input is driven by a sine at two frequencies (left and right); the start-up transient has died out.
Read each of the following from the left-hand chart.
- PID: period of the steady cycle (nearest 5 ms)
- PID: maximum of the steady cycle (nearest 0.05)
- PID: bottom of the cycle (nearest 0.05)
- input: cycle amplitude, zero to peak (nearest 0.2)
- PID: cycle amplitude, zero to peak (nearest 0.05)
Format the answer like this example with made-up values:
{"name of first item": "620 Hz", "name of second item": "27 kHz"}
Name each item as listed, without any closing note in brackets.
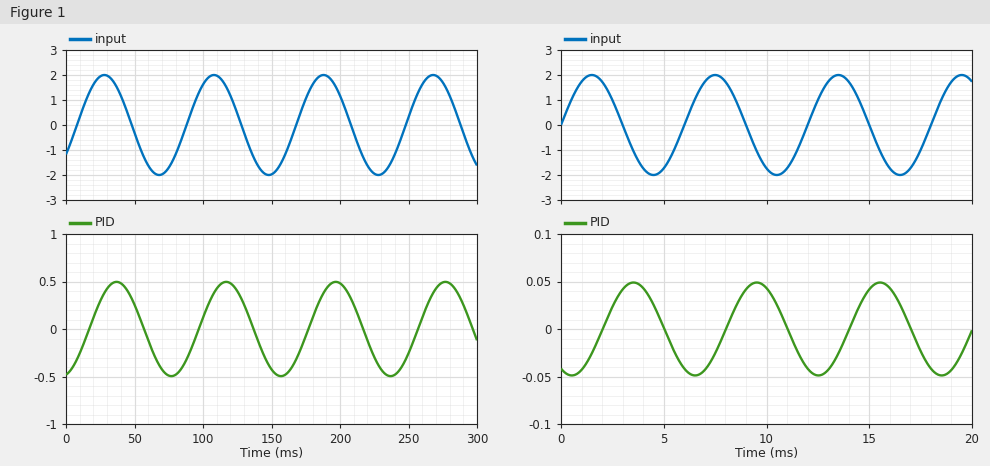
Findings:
{"PID: period of the steady cycle": "80 ms", "PID: maximum of the steady cycle": "0.50", "PID: bottom of the cycle": "-0.50", "input: cycle amplitude, zero to peak": "2.0", "PID: cycle amplitude, zero to peak": "0.50"}
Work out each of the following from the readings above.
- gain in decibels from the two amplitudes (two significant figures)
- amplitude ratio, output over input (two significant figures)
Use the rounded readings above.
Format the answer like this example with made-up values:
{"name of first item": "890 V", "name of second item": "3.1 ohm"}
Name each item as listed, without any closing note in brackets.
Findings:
{"gain in decibels from the two amplitudes": "-12 dB", "amplitude ratio, output over input": "0.25"}
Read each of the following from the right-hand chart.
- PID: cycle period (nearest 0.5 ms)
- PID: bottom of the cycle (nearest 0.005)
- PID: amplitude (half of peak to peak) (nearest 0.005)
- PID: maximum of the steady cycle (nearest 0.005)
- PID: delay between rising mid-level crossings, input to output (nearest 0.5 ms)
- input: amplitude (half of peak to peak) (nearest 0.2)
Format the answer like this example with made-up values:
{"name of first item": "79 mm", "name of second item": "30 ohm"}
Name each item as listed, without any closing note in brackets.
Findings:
{"PID: cycle period": "6.0 ms", "PID: bottom of the cycle": "-0.050", "PID: amplitude (half of peak to peak)": "0.050", "PID: maximum of the steady cycle": "0.050", "PID: delay between rising mid-level crossings, input to output": "2.0 ms", "input: amplitude (half of peak to peak)": "2.0"}
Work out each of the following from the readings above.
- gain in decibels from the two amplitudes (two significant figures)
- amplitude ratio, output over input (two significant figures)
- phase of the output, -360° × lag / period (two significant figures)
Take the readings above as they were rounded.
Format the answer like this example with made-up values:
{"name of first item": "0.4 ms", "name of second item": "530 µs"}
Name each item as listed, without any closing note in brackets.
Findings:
{"gain in decibels from the two amplitudes": "-32 dB", "amplitude ratio, output over input": "0.025", "phase of the output, -360° × lag / period": "-120°"}
